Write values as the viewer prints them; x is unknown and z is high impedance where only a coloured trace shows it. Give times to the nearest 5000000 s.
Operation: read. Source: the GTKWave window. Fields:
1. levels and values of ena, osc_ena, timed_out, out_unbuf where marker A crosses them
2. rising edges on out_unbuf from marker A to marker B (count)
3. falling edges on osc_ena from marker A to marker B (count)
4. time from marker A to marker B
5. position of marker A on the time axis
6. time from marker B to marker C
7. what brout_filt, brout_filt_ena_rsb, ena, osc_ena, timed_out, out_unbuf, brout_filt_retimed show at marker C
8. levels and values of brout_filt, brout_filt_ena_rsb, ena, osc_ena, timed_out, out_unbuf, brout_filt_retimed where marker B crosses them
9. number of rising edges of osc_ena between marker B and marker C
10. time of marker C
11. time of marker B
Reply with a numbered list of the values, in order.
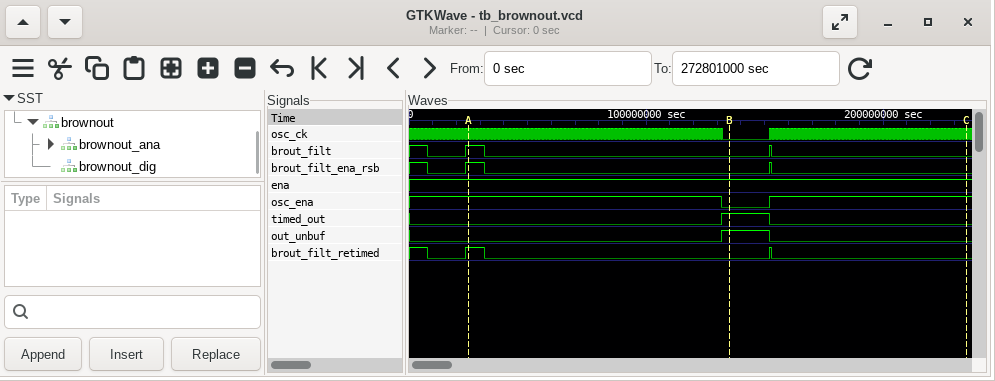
1. ena=1, osc_ena=1, timed_out=0, out_unbuf=0
2. 1
3. 1
4. 110000000 s
5. 25000000 s
6. 100000000 s
7. brout_filt=0, brout_filt_ena_rsb=0, ena=1, osc_ena=1, timed_out=0, out_unbuf=0, brout_filt_retimed=0
8. brout_filt=0, brout_filt_ena_rsb=0, ena=1, osc_ena=0, timed_out=1, out_unbuf=1, brout_filt_retimed=0
9. 1
10. 235000000 s
11. 135000000 s
